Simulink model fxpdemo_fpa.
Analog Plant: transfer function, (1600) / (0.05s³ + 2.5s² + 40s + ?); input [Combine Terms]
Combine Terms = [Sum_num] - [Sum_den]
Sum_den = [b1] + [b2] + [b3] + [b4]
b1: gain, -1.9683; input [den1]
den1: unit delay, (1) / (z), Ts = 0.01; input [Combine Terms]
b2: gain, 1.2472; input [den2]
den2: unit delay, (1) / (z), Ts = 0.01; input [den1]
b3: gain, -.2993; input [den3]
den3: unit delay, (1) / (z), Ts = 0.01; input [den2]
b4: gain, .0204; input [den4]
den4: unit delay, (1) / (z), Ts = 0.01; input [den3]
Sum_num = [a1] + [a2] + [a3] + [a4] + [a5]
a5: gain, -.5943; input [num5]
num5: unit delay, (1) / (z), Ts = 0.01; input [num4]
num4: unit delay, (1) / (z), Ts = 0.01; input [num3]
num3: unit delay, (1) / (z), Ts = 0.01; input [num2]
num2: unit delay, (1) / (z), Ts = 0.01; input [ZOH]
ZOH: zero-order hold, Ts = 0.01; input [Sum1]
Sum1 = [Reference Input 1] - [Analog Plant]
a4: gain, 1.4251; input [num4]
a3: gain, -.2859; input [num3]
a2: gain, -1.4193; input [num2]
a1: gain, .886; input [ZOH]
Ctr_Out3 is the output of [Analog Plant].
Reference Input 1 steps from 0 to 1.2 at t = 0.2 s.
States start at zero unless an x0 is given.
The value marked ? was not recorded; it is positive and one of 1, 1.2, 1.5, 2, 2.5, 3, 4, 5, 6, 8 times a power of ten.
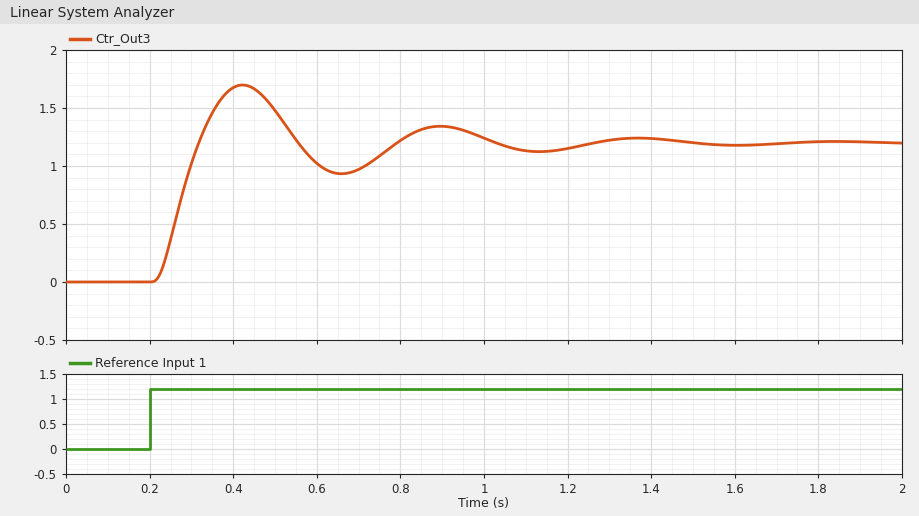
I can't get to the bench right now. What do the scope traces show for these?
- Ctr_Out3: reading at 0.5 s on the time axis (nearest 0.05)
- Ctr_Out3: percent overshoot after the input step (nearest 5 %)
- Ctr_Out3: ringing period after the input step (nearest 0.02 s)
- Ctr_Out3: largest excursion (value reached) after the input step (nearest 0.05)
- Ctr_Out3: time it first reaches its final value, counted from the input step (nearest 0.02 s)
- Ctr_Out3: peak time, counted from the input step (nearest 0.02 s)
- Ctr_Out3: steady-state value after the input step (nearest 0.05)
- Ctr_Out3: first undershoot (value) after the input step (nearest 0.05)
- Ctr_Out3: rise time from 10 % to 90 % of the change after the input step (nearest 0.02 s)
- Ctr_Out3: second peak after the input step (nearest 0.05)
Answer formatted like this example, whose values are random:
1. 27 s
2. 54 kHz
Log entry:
1. 1.50
2. 40 %
3. 0.48 s
4. 1.70
5. 0.12 s
6. 0.22 s
7. 1.20
8. 0.95
9. 0.08 s
10. 1.35
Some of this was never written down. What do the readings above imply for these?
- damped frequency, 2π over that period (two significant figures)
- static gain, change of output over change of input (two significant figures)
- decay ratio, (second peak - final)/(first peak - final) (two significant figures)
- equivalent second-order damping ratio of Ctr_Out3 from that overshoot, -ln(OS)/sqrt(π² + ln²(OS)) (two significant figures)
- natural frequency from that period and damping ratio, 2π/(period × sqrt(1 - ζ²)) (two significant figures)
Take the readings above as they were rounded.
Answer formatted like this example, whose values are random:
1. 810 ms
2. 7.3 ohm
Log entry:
1. 13 rad/s
2. 1.0
3. 0.30
4. 0.28
5. 14 rad/s
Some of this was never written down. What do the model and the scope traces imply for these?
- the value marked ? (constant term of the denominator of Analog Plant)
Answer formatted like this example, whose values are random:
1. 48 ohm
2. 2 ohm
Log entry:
1. 200
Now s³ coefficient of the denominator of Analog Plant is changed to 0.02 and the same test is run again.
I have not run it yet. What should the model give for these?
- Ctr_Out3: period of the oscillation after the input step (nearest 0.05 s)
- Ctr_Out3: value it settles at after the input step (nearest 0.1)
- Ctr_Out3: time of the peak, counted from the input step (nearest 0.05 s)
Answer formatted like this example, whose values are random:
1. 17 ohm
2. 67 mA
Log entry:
1. 0.50 s
2. 1.2
3. 0.25 s
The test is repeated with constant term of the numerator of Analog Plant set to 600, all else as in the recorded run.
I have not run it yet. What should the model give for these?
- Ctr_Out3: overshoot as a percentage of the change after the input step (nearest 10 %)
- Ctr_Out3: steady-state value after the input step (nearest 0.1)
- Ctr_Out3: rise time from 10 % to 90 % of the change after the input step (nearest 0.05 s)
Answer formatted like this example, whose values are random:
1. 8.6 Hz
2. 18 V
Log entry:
1. 30 %
2. 1.2
3. 0.15 s
